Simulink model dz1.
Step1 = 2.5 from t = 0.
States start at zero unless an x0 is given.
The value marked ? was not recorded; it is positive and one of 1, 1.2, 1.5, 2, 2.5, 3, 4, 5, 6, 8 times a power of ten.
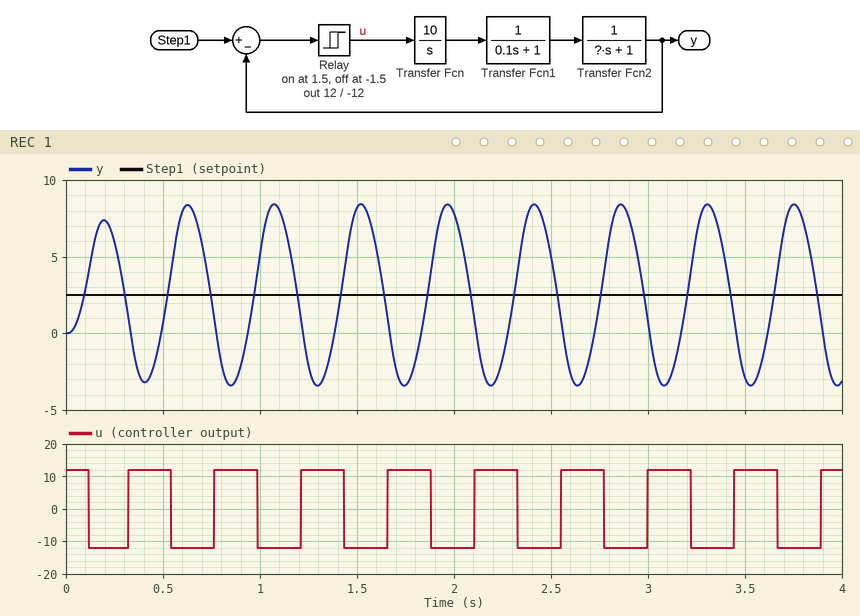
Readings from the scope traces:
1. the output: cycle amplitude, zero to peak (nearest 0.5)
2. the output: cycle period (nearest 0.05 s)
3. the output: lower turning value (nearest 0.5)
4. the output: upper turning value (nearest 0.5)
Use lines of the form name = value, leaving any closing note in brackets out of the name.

the output: cycle amplitude, zero to peak = 6.0
the output: cycle period = 0.45 s
the output: lower turning value = -3.5
the output: upper turning value = 8.5
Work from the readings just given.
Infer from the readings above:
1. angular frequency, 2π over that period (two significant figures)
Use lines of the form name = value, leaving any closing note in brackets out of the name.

angular frequency, 2π over that period = 14 rad/s
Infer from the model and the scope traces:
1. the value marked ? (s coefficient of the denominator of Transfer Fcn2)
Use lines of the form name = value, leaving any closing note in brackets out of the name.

the value marked ? = 0.025
